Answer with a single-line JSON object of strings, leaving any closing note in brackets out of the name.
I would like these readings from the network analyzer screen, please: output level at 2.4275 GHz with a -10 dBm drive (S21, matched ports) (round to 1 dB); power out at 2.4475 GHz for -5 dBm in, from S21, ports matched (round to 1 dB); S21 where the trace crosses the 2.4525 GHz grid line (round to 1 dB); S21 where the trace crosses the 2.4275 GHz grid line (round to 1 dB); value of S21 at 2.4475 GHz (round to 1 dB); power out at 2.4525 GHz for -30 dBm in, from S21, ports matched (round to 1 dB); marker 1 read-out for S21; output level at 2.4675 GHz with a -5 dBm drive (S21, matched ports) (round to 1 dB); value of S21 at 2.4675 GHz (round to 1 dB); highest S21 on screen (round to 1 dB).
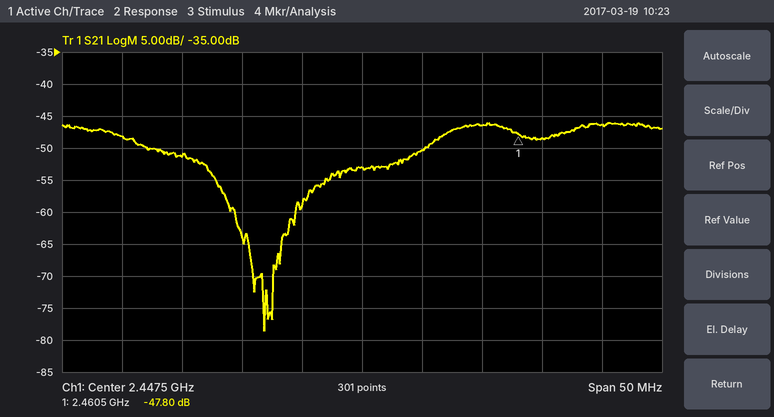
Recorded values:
{"output level at 2.4275 GHz with a -10 dBm drive (S21, matched ports)": "-58 dBm", "power out at 2.4475 GHz for -5 dBm in, from S21, ports matched": "-58 dBm", "S21 where the trace crosses the 2.4525 GHz grid line": "-50 dB", "S21 where the trace crosses the 2.4275 GHz grid line": "-48 dB", "value of S21 at 2.4475 GHz": "-53 dB", "power out at 2.4525 GHz for -30 dBm in, from S21, ports matched": "-80 dBm", "marker 1 read-out for S21": "-47.80 dB", "output level at 2.4675 GHz with a -5 dBm drive (S21, matched ports)": "-51 dBm", "value of S21 at 2.4675 GHz": "-46 dB", "highest S21 on screen": "-46 dB"}
